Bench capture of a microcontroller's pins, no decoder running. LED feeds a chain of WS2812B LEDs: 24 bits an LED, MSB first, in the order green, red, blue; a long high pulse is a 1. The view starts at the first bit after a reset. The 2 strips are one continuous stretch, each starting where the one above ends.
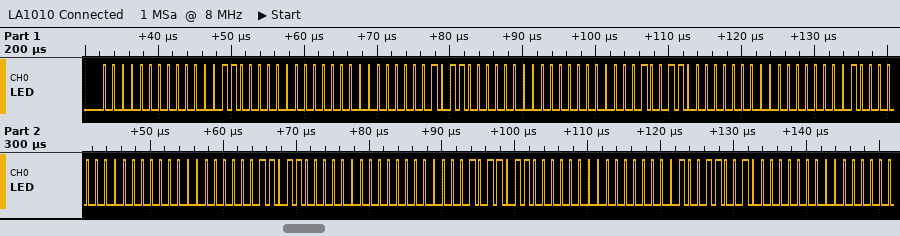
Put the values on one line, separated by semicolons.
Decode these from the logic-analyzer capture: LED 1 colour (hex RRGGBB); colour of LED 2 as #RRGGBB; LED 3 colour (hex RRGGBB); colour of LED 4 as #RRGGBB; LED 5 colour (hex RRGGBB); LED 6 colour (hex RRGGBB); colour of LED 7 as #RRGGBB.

#060000; #0B0000; #130000; #200000; #360000; #5B0000; #990000
